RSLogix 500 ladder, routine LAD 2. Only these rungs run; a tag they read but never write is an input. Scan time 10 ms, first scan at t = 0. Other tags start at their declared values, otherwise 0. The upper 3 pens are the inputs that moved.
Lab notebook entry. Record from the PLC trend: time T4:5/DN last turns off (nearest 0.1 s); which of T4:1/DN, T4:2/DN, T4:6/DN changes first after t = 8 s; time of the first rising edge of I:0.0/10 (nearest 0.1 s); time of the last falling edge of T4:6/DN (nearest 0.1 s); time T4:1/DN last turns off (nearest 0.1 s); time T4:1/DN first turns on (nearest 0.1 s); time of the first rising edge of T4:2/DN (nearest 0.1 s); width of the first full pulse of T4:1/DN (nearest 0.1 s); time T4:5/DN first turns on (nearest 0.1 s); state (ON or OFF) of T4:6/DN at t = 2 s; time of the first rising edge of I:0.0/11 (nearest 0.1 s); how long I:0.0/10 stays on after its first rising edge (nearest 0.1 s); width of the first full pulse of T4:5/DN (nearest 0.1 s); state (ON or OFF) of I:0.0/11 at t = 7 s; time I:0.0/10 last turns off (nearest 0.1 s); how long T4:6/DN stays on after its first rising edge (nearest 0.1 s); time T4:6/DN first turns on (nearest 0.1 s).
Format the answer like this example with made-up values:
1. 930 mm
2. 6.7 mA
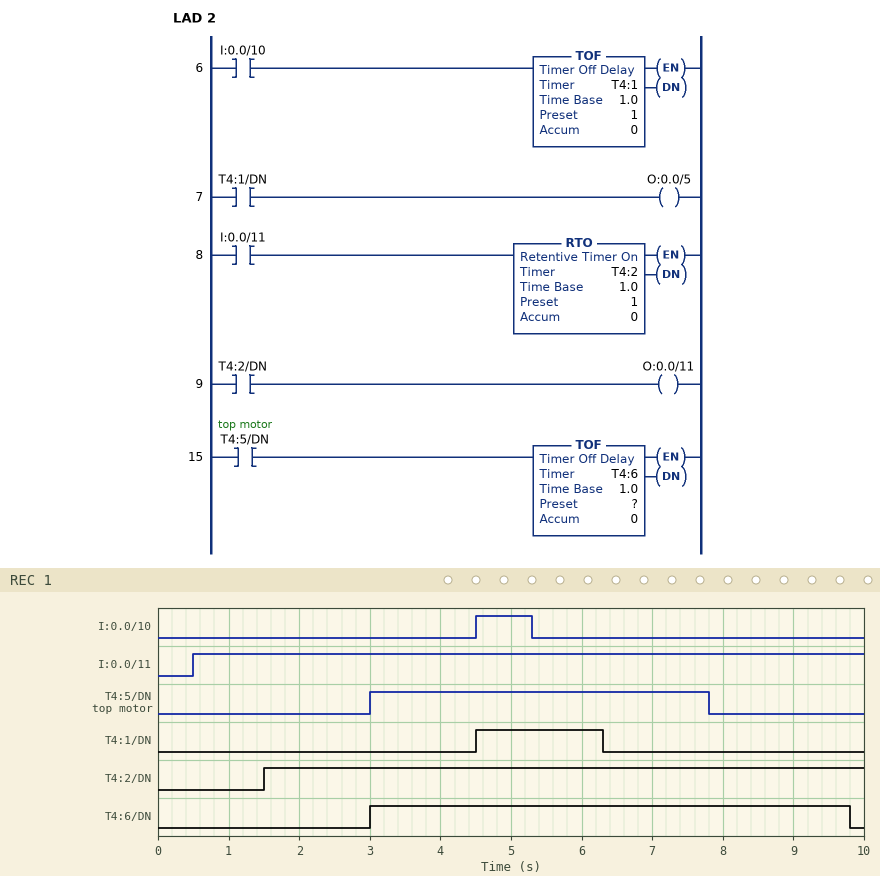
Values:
1. 7.8 s
2. T4:6/DN
3. 4.5 s
4. 9.8 s
5. 6.3 s
6. 4.5 s
7. 1.5 s
8. 1.8 s
9. 3.0 s
10. OFF
11. 0.5 s
12. 0.8 s
13. 4.8 s
14. ON
15. 5.3 s
16. 6.8 s
17. 3.0 s
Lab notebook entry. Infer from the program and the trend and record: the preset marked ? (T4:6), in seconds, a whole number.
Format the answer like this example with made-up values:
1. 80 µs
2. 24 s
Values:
1. 2 s
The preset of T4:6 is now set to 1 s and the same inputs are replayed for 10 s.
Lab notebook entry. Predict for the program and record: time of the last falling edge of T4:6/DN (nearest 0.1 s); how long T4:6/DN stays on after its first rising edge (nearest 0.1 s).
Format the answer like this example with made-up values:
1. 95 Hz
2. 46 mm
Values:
1. 8.8 s
2. 5.8 s
